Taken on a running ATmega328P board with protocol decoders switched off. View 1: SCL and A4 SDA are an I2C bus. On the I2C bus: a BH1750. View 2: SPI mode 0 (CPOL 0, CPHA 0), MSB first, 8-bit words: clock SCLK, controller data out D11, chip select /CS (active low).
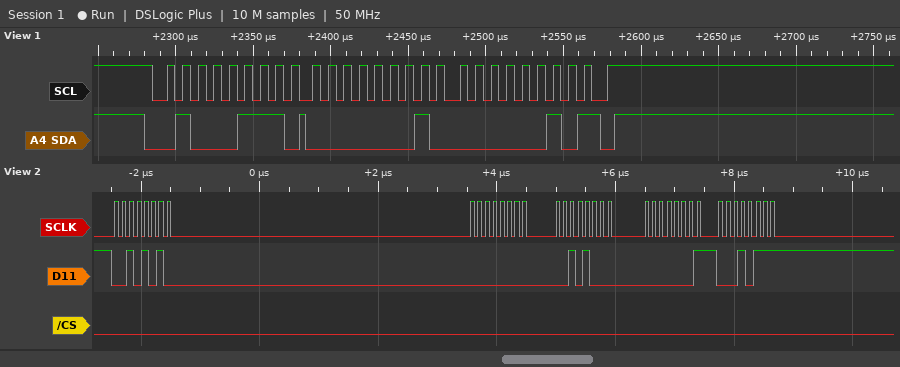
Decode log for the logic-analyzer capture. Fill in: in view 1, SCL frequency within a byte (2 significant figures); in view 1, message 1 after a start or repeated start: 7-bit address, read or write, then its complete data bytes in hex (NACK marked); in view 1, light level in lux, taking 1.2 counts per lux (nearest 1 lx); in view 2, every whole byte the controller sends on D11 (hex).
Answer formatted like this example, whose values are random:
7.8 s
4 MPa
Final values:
100 kHz
0x23 read: 01 02 NACK
215 lx
2A 00 28 01 17
